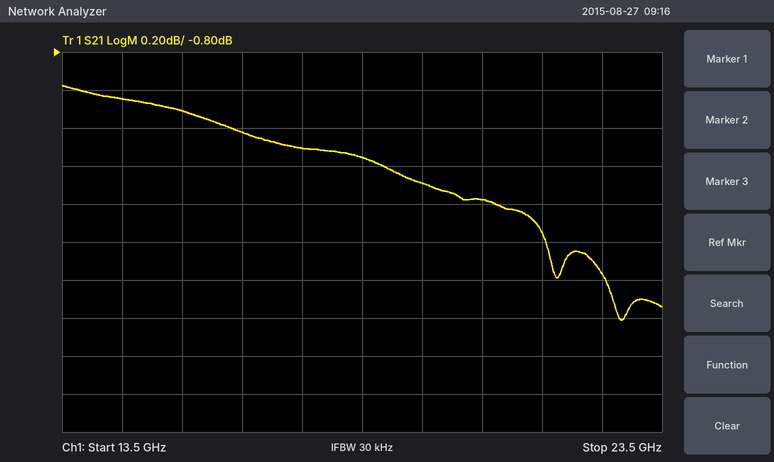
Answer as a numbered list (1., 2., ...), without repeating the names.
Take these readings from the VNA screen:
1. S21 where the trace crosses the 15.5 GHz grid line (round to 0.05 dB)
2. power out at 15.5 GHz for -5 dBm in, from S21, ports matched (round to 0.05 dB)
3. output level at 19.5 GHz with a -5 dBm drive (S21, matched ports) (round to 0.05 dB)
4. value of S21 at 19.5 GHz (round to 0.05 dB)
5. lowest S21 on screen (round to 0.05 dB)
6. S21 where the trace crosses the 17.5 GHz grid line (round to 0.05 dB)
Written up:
1. -1.10 dB
2. -6.10 dBm
3. -6.50 dBm
4. -1.50 dB
5. -2.20 dB
6. -1.30 dB
